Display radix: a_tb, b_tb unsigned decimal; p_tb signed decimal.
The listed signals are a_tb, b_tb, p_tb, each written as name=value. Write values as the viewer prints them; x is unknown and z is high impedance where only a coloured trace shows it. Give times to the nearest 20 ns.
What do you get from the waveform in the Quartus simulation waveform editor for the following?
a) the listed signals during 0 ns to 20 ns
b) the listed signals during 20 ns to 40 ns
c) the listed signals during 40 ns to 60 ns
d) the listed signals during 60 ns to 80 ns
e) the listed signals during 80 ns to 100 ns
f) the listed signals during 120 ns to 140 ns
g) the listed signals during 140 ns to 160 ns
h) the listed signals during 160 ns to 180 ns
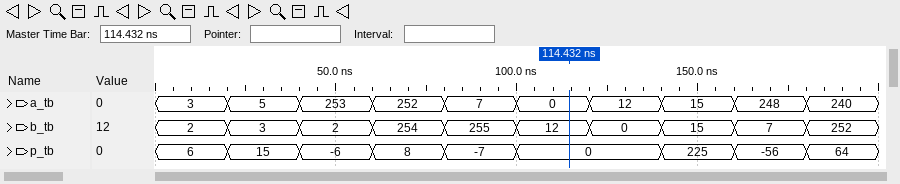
a_tb=3, b_tb=2, p_tb=6
a_tb=5, b_tb=3, p_tb=15
a_tb=253, b_tb=2, p_tb=-6
a_tb=252, b_tb=254, p_tb=8
a_tb=7, b_tb=255, p_tb=-7
a_tb=12, b_tb=0, p_tb=0
a_tb=15, b_tb=15, p_tb=225
a_tb=248, b_tb=7, p_tb=-56
